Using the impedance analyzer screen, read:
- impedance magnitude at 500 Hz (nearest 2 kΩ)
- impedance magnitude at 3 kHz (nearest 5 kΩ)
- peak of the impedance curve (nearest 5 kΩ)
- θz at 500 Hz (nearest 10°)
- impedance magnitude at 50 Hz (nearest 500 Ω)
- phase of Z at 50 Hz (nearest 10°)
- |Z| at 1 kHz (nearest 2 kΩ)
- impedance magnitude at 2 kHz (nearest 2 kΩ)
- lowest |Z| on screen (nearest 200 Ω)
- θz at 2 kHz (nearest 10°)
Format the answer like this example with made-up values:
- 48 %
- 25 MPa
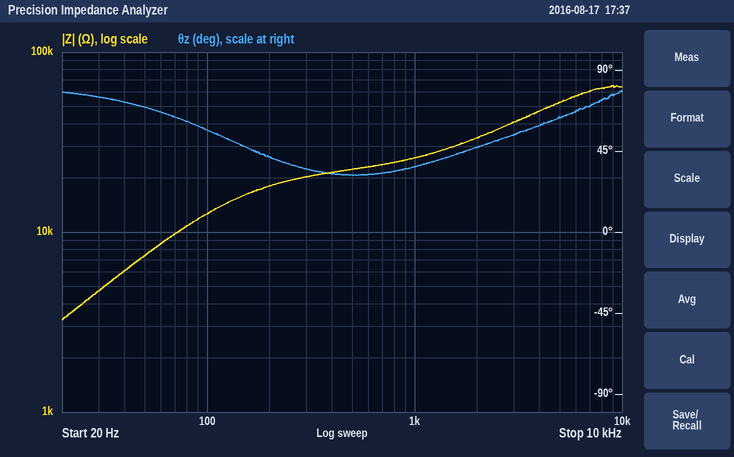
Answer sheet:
- 22 kΩ
- 40 kΩ
- 65 kΩ
- 30°
- 7.5 kΩ
- 70°
- 26 kΩ
- 34 kΩ
- 3.2 kΩ
- 50°
